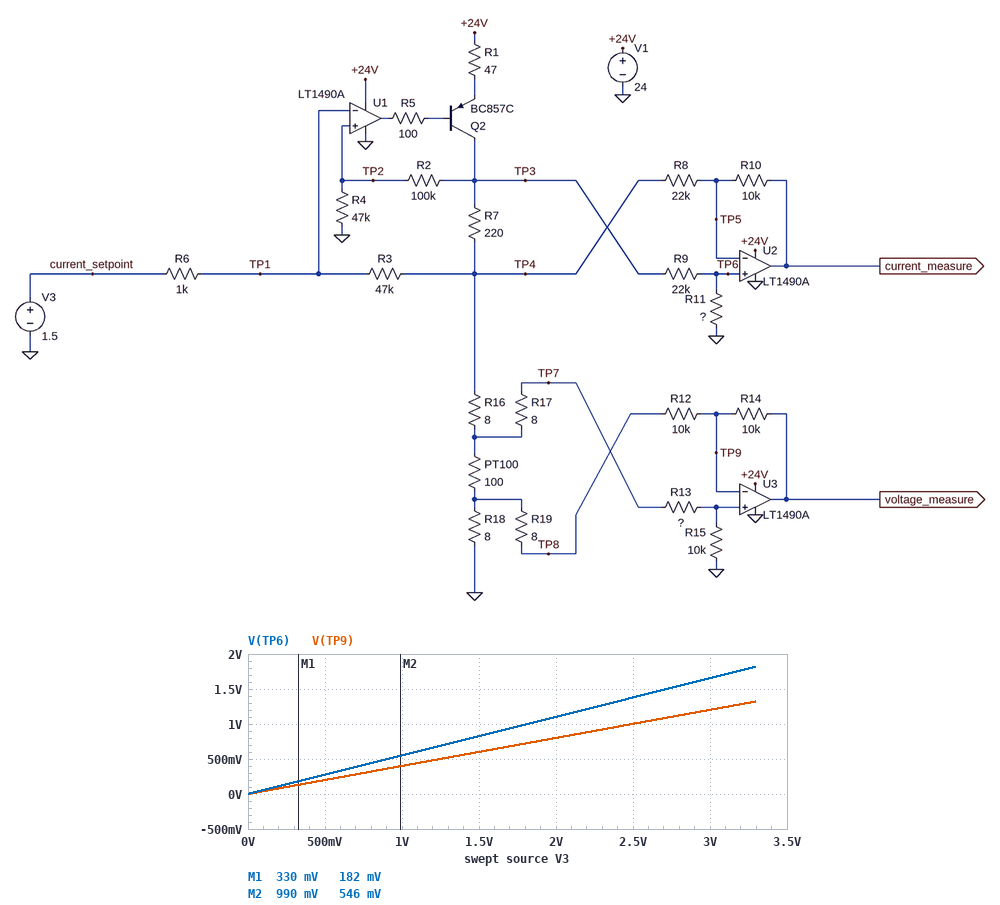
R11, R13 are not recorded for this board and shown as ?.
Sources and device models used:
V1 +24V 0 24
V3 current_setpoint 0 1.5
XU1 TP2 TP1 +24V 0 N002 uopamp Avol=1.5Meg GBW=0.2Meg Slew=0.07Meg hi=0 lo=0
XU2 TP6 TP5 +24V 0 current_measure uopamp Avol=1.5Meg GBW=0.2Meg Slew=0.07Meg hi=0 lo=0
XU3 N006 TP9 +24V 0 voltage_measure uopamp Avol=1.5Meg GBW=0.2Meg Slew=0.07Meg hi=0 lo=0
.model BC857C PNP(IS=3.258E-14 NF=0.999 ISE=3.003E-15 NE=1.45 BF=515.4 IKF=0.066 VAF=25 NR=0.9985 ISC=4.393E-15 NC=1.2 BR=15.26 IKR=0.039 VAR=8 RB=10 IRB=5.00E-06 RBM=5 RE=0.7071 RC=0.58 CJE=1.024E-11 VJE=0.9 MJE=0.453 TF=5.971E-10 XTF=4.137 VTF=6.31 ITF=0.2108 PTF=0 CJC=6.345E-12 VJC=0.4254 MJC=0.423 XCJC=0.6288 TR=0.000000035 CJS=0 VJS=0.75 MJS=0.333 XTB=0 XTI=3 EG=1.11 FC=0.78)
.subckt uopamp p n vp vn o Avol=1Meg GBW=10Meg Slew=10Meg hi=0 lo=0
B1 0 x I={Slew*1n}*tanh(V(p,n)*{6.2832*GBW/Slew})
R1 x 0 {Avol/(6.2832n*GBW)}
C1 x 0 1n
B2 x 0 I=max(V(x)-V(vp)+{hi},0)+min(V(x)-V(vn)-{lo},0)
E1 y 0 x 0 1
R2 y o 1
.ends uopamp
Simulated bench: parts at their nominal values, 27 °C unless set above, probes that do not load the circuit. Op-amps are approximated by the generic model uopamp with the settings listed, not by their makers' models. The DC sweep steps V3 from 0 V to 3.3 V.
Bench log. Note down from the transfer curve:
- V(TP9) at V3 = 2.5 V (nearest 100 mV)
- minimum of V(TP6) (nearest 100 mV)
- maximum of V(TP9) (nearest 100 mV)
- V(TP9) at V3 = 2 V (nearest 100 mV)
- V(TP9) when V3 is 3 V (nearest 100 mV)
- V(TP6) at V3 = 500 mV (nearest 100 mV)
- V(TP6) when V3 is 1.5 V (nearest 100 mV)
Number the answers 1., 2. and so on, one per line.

1. 1.0 V
2. 0 V
3. 1.3 V
4. 800 mV
5. 1.2 V
6. 300 mV
7. 800 mV
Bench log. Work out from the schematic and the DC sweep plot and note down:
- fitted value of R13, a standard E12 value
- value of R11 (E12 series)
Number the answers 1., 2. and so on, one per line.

1. 15 kΩ
2. 4.7 kΩ
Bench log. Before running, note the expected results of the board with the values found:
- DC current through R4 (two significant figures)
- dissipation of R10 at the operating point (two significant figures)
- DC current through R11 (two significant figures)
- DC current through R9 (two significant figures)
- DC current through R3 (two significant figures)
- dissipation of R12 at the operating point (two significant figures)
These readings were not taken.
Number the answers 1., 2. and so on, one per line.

1. 32 µA
2. 13 µW
3. 180 µA
4. 180 µA
5. 2.4 µA
6. 24 µW
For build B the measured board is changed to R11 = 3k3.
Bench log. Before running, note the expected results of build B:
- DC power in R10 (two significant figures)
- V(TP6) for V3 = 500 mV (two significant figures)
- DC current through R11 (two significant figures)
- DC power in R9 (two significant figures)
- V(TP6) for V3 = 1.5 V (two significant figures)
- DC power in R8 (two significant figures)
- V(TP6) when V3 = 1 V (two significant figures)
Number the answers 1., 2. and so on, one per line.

1. 21 µW
2. 200 mV
3. 190 µA
4. 760 µW
5. 610 mV
6. 46 µW
7. 410 mV
